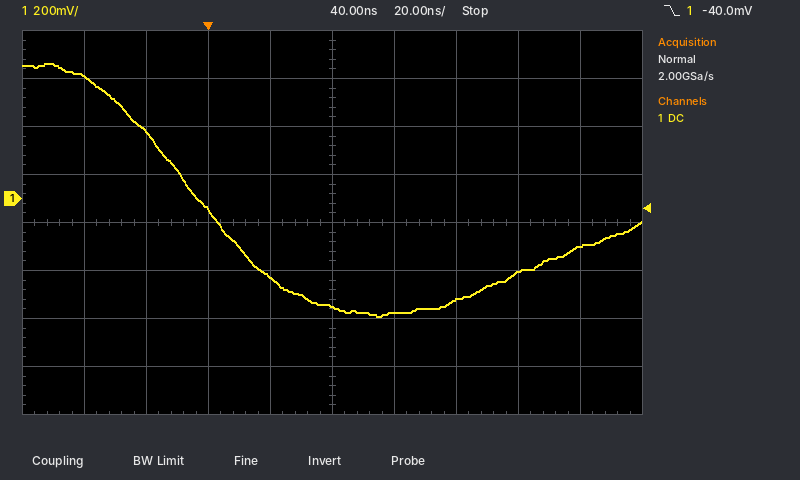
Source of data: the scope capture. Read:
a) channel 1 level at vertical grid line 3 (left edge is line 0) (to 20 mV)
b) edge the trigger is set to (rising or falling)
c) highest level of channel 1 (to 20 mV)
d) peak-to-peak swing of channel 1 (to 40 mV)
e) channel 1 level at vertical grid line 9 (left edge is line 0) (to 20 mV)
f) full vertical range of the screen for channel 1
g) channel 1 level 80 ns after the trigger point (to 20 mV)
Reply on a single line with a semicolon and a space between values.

-40 mV; falling; 560 mV; 1.04 V; -200 mV; 1.6 V; -420 mV
